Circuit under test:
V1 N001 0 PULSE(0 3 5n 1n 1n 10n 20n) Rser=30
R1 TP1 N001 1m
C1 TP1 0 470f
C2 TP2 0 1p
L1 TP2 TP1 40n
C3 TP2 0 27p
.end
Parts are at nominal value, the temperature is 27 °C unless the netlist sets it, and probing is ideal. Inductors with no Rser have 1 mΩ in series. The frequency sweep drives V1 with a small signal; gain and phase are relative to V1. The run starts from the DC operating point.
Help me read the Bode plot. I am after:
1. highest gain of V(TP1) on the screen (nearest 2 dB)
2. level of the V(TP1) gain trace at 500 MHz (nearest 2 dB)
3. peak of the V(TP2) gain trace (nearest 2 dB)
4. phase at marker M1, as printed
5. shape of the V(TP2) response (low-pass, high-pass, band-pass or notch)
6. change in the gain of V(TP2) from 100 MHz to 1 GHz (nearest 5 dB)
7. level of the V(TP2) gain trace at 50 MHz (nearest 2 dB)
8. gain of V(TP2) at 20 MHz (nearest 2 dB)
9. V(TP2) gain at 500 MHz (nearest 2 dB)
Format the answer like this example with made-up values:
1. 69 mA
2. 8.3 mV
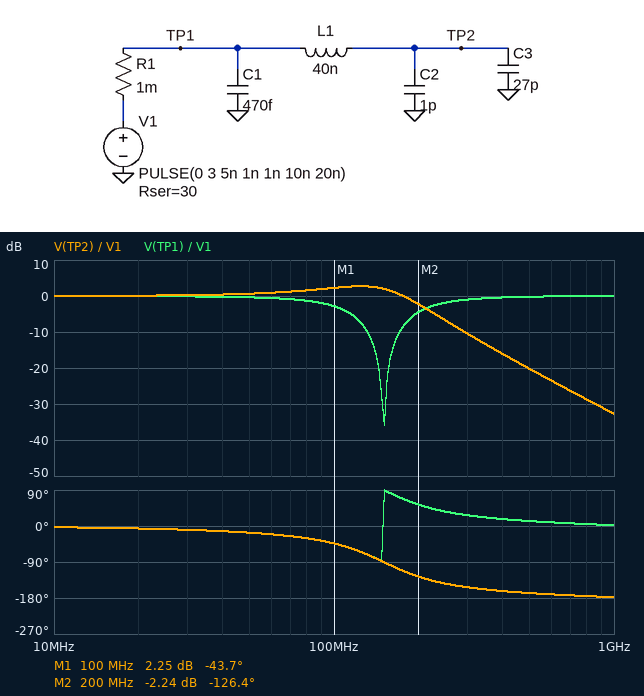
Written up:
1. 0 dB
2. 0 dB
3. 2 dB
4. -43.7 deg
5. low-pass
6. -35 dB
7. 0 dB
8. 0 dB
9. -20 dB
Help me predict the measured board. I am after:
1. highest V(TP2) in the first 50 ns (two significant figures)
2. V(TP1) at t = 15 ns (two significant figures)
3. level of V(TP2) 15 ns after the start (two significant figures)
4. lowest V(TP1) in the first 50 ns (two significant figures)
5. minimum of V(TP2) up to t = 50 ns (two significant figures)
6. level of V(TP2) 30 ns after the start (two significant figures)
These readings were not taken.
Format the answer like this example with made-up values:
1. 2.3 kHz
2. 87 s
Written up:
1. 3.7 V
2. 2.9 V
3. 3.0 V
4. -360 mV
5. -750 mV
6. 3.6 V
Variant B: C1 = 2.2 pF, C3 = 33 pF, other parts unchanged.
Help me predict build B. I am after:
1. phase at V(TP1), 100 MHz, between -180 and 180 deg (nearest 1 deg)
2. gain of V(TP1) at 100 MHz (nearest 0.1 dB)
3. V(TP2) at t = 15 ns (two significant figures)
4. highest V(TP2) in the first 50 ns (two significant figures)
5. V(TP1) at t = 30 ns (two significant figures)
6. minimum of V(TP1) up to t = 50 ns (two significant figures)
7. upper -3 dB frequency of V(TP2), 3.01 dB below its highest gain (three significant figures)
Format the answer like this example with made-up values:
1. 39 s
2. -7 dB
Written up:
1. -55 deg
2. -4.8 dB
3. 2.9 V
4. 3.6 V
5. 3.1 V
6. -310 mV
7. 166 MHz
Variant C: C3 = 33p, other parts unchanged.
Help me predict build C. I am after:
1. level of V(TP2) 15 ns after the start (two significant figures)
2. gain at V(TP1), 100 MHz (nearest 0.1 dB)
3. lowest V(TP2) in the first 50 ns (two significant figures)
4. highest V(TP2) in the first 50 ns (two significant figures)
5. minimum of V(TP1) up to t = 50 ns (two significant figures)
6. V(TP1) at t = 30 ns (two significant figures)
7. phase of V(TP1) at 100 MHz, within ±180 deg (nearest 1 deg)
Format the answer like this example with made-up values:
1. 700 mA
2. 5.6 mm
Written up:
1. 2.9 V
2. -4.7 dB
3. -630 mV
4. 3.6 V
5. -320 mV
6. 3.1 V
7. -54 deg
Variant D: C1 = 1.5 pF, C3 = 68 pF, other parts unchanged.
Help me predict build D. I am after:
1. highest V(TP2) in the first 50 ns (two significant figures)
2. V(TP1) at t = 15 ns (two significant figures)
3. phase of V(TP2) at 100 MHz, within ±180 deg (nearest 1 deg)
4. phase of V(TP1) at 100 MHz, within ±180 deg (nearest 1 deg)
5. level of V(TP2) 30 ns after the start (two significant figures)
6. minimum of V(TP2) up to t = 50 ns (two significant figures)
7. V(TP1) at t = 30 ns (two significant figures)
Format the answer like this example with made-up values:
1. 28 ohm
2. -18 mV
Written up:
1. 3.2 V
2. 3.1 V
3. -94 deg
4. 86 deg
5. 2.9 V
6. -230 mV
7. 2.2 V
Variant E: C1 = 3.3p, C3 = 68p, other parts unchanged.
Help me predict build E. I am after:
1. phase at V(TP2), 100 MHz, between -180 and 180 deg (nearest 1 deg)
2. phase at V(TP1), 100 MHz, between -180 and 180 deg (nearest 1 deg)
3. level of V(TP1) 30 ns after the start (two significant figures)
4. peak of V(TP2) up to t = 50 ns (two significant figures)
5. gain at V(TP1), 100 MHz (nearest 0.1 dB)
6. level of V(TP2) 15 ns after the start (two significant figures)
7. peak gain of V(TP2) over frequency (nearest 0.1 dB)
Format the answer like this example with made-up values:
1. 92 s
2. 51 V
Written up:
1. -94 deg
2. 86 deg
3. 2.2 V
4. 3.2 V
5. -23.2 dB
6. 3.1 V
7. 0.1 dB
